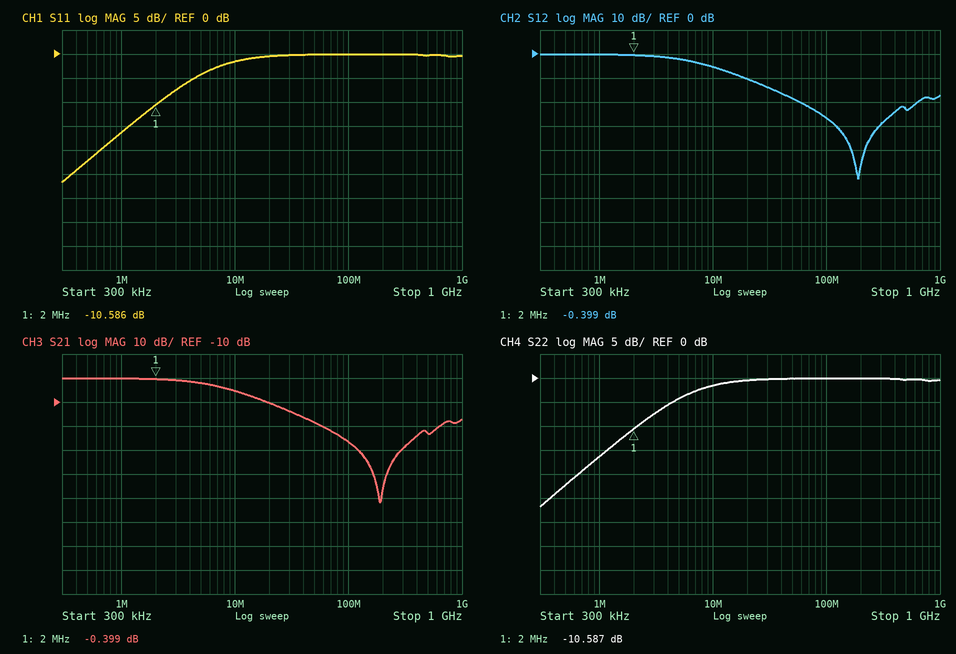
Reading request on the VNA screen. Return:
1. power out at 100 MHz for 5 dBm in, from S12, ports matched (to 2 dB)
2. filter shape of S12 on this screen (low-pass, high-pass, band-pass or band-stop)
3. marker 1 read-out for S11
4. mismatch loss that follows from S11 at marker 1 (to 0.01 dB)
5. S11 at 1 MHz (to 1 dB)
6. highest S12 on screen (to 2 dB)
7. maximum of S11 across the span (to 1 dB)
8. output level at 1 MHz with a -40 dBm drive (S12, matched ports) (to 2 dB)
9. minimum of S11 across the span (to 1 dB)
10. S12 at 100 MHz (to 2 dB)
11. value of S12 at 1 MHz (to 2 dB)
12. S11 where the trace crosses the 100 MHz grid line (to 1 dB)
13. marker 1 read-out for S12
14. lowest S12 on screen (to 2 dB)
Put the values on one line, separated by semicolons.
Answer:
-22 dBm; low-pass; -10.586 dB; 0.40 dB; -16 dB; 0 dB; 0 dB; -40 dBm; -27 dB; -26 dB; 0 dB; 0 dB; -0.399 dB; -52 dB
